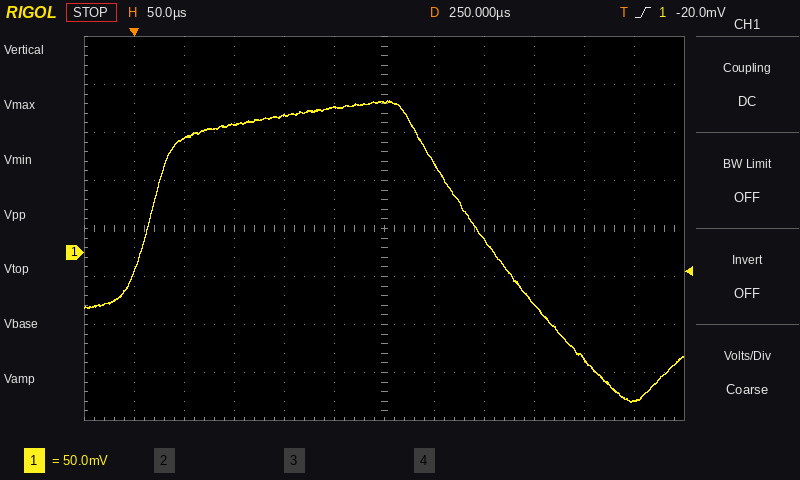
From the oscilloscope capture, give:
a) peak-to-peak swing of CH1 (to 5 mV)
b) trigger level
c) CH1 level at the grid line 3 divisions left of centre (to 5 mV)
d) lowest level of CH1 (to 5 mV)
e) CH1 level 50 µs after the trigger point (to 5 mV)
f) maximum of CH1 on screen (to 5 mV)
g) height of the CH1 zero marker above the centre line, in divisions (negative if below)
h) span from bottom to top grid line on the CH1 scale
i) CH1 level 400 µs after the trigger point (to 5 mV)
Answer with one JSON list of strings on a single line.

["315 mV", "-20.0 mV", "135 mV", "-155 mV", "120 mV", "160 mV", "-0.5 div", "400 mV", "-55 mV"]
